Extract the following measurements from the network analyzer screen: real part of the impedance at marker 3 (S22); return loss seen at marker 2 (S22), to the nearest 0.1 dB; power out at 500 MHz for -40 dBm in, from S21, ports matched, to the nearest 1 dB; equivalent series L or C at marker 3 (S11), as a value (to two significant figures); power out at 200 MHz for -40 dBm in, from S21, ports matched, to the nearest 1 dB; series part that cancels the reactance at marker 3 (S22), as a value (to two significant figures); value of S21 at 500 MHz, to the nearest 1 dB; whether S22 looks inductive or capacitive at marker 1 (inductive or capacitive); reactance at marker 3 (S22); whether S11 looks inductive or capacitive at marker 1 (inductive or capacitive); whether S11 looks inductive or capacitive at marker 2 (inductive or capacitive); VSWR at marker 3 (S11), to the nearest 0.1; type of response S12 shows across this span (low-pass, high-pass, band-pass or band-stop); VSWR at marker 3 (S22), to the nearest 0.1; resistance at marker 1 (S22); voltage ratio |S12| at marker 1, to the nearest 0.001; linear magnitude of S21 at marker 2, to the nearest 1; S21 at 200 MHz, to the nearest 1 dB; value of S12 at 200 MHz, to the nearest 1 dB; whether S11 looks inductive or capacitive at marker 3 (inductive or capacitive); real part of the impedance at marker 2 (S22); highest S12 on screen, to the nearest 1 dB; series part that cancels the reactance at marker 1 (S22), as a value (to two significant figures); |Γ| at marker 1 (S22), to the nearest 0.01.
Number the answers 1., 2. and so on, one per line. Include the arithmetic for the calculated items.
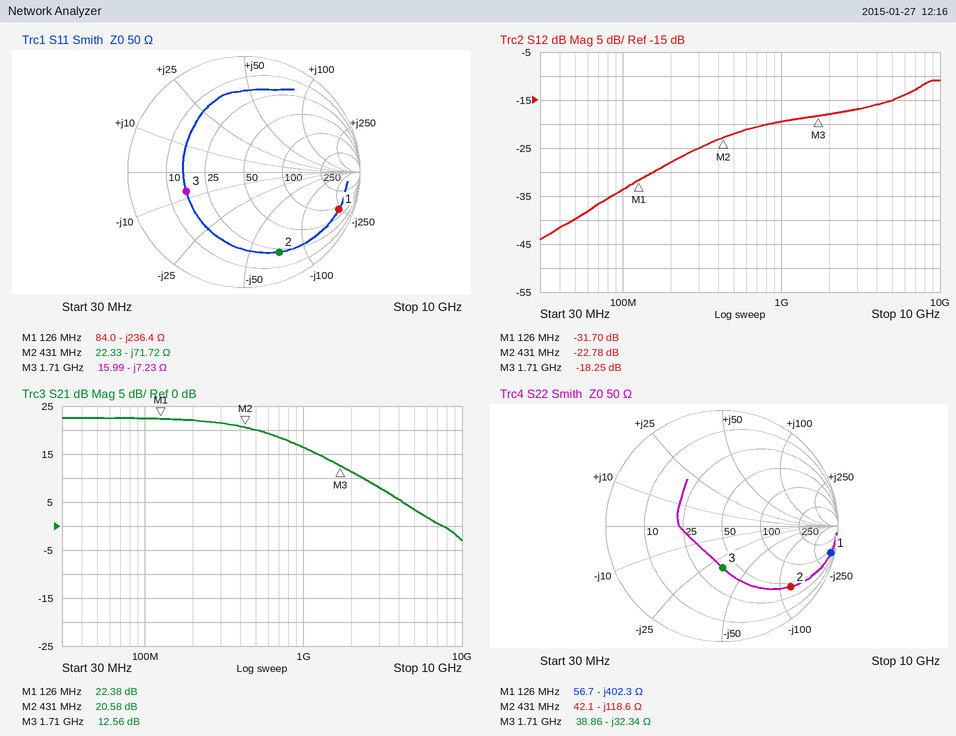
1. 38.86 Ω
2. 2.0 dB
3. -40 dBm + (20 dB) = -20 dBm
4. C = 1/(2π × 1.71 GHz × 7.23 Ω) ≈ 13 pF
5. -40 dBm + (22 dB) = -18 dBm
6. L = 32.34 Ω/(2π × 1.71 GHz) ≈ 3.0 nH
7. 20 dB
8. capacitive
9. -32.34 Ω
10. capacitive
11. capacitive
12. 3.2
13. high-pass
14. 2.1
15. 56.7 Ω
16. 10^(-31.7/20) ≈ 0.026
17. 10^(20.58/20) ≈ 11
18. 22 dB
19. -28 dB
20. capacitive
21. 42.1 Ω
22. -11 dB
23. L = 402.3 Ω/(2π × 126 MHz) ≈ 508 nH, so 510 nH to two significant figures
24. 0.97
